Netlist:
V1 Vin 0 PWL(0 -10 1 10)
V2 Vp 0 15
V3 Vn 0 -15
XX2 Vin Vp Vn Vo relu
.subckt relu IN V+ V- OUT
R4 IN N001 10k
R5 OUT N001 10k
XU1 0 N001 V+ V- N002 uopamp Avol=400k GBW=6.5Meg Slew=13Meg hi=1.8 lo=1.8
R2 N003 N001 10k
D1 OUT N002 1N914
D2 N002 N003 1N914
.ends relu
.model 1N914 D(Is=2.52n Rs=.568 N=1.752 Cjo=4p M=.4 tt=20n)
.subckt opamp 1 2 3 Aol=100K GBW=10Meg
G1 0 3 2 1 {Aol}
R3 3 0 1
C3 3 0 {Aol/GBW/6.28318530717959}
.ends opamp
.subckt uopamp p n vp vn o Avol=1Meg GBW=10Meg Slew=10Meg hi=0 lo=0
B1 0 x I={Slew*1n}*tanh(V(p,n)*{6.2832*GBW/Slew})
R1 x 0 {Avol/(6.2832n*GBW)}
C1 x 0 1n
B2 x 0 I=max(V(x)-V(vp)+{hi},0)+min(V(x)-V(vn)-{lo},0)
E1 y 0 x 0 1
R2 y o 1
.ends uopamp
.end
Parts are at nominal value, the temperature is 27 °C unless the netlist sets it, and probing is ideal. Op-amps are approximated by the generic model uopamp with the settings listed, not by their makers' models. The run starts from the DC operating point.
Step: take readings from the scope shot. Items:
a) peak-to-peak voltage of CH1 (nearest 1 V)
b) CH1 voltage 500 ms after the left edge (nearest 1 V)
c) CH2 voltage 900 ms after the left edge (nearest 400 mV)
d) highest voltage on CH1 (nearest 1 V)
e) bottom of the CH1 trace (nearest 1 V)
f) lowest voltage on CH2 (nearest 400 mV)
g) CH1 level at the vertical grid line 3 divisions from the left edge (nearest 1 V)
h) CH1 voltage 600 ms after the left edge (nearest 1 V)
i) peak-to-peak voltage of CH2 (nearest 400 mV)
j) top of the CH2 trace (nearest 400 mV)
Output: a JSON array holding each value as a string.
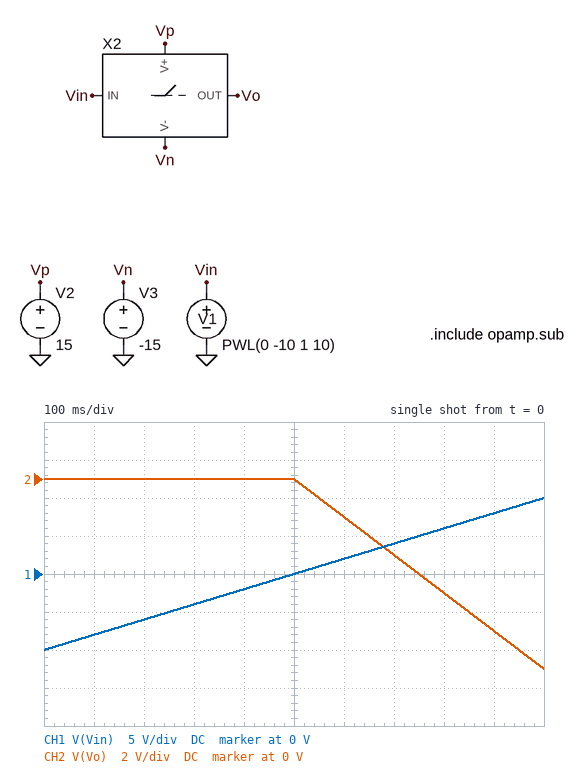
["20 V", "0 V", "-8.0 V", "10 V", "-10 V", "-10.0 V", "-4 V", "2 V", "10.0 V", "0 V"]
